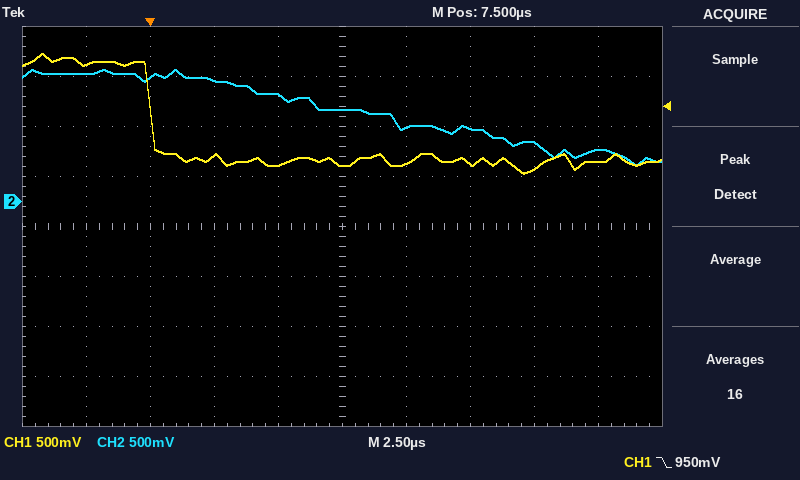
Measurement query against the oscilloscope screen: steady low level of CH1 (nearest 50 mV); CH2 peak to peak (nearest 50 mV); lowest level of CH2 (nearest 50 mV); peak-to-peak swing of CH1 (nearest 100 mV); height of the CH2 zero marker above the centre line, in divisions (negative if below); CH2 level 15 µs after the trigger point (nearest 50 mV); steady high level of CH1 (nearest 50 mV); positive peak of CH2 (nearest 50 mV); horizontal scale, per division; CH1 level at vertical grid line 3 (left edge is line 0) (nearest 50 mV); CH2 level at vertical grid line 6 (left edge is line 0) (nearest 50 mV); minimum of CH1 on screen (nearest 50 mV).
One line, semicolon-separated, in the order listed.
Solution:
400 mV; 950 mV; 350 mV; 1.20 V; +0.5 div; 600 mV; 1.40 V; 1.30 V; 2.5 µs; 450 mV; 750 mV; 300 mV
